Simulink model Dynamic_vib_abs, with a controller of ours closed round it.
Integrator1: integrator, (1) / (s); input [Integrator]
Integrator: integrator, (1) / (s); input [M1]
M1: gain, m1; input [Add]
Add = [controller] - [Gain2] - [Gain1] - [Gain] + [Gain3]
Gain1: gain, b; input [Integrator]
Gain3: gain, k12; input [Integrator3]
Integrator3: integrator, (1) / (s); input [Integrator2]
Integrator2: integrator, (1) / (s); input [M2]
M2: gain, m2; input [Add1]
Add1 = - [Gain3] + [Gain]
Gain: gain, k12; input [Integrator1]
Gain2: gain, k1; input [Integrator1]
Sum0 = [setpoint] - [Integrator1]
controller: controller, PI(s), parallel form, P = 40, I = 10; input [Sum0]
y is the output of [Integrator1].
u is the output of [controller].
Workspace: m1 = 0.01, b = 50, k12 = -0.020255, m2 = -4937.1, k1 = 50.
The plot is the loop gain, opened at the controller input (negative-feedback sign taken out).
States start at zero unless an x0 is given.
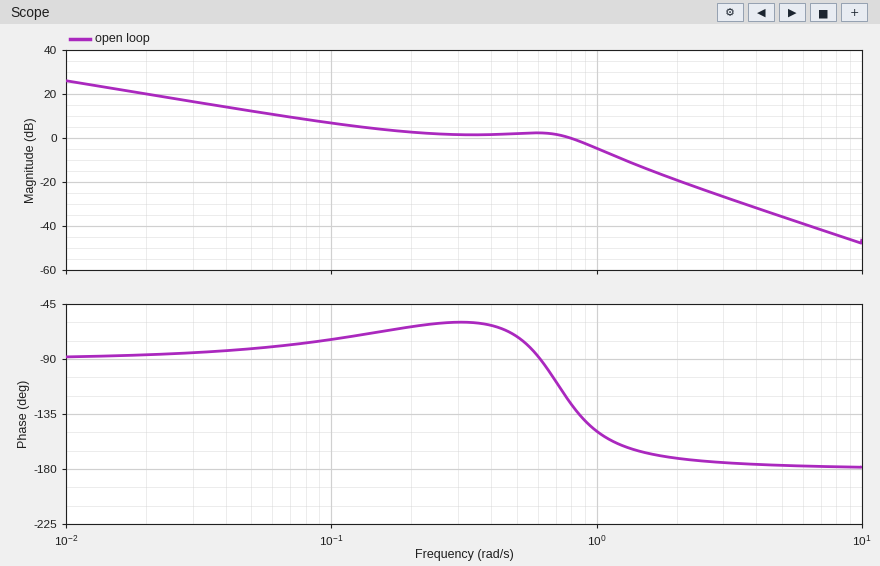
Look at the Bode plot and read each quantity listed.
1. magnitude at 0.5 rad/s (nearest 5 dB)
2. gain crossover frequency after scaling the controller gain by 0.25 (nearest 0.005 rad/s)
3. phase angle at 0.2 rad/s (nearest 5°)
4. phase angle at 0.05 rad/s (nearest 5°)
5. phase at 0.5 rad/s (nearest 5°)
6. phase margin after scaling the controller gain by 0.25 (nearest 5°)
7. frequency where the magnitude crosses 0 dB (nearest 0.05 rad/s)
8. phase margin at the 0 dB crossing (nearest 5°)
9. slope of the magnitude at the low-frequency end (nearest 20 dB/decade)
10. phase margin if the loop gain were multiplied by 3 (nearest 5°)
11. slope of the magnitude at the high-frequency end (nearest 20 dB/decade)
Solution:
0 dB
0.050 rad/s
-65°
-80°
-70°
100°
0.80 rad/s
55°
-20 dB/decade
20°
-40 dB/decade
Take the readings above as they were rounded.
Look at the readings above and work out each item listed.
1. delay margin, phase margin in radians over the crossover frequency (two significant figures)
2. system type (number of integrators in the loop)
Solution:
1.2 s
1
